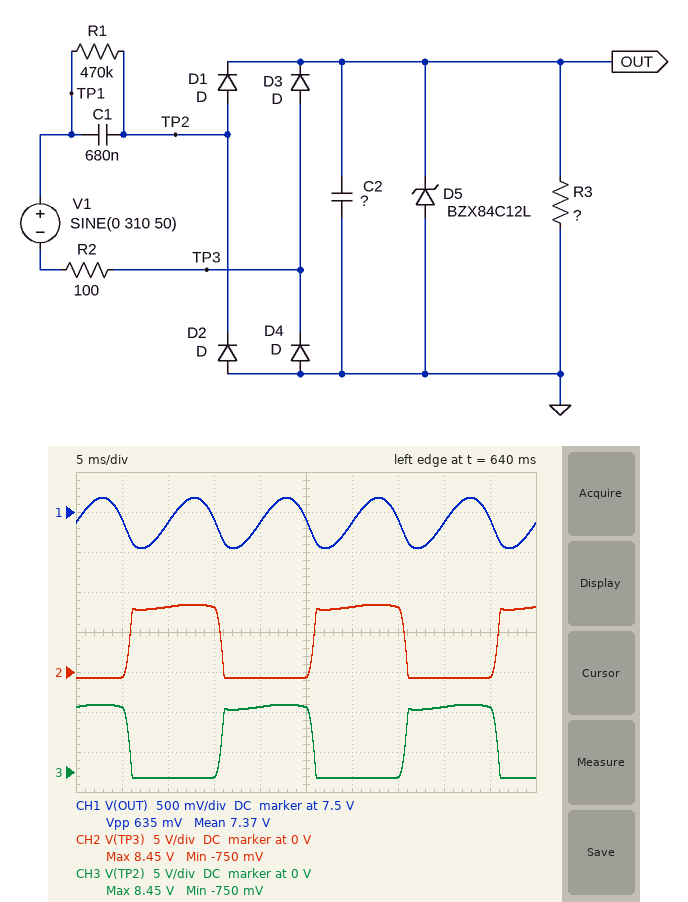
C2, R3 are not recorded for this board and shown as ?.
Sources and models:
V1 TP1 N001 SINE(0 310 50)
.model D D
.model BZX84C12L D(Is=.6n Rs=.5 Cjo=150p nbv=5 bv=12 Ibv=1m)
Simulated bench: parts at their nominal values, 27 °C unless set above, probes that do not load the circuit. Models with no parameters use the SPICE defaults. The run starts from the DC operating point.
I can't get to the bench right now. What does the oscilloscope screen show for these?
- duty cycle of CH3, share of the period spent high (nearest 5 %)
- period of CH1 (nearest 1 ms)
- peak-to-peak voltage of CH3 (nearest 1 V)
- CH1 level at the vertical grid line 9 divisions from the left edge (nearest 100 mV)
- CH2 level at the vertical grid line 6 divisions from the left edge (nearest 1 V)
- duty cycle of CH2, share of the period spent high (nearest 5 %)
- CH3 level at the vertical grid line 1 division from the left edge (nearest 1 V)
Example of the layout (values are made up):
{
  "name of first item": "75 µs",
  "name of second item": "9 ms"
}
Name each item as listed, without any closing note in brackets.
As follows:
{
  "duty cycle of CH3, share of the period spent high": "50 %",
  "period of CH1": "10 ms",
  "peak-to-peak voltage of CH3": "9 V",
  "CH1 level at the vertical grid line 9 divisions from the left edge": "7.4 V",
  "CH2 level at the vertical grid line 6 divisions from the left edge": "8 V",
  "duty cycle of CH2, share of the period spent high": "50 %",
  "CH3 level at the vertical grid line 1 division from the left edge": "8 V"
}
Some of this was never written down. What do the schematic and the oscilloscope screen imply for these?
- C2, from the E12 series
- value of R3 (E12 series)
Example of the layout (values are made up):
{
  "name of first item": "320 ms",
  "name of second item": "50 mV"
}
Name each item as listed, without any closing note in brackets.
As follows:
{
  "C2, from the E12 series": "150 µF",
  "value of R3": "180 Ω"
}
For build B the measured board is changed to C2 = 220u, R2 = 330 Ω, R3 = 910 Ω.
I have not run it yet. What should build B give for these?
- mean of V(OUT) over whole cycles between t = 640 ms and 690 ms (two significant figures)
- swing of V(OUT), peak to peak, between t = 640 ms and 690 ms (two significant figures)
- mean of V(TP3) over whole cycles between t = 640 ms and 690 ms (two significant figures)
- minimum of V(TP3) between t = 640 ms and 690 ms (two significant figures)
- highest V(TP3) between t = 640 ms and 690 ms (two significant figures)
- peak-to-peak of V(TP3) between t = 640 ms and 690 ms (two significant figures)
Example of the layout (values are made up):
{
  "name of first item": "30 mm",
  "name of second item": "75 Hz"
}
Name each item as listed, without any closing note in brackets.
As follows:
{
  "mean of V(OUT) over whole cycles between t = 640 ms and 690 ms": "12 V",
  "swing of V(OUT), peak to peak, between t = 640 ms and 690 ms": "320 mV",
  "mean of V(TP3) over whole cycles between t = 640 ms and 690 ms": "6.2 V",
  "minimum of V(TP3) between t = 640 ms and 690 ms": "-760 mV",
  "highest V(TP3) between t = 640 ms and 690 ms": "13 V",
  "peak-to-peak of V(TP3) between t = 640 ms and 690 ms": "14 V"
}
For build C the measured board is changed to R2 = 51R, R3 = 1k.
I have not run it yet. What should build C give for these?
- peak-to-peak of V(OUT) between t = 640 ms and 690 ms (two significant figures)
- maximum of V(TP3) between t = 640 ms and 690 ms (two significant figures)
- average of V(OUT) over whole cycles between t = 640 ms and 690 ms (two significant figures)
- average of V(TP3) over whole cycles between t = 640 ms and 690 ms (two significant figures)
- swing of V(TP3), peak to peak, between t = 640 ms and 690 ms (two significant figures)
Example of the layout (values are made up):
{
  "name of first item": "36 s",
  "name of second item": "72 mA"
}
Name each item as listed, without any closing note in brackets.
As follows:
{
  "peak-to-peak of V(OUT) between t = 640 ms and 690 ms": "400 mV",
  "maximum of V(TP3) between t = 640 ms and 690 ms": "13 V",
  "average of V(OUT) over whole cycles between t = 640 ms and 690 ms": "12 V",
  "average of V(TP3) over whole cycles between t = 640 ms and 690 ms": "6.2 V",
  "swing of V(TP3), peak to peak, between t = 640 ms and 690 ms": "14 V"
}
